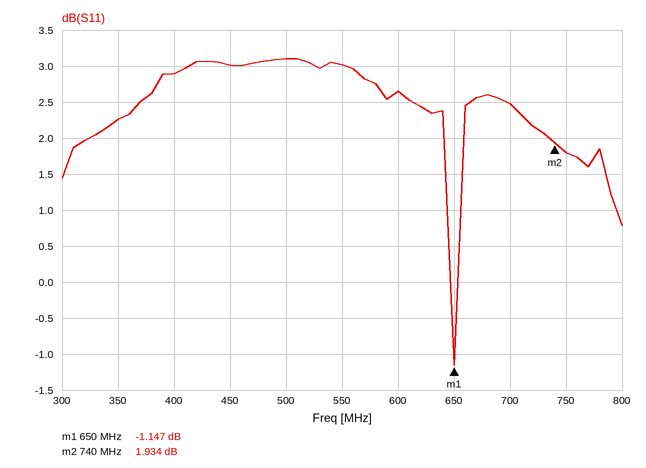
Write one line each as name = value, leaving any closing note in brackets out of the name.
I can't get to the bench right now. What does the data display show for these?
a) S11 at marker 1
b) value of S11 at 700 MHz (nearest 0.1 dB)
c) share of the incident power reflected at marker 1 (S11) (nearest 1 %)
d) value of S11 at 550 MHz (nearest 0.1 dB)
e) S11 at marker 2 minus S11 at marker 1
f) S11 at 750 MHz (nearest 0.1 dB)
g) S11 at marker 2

S11 at marker 1 = -1.147 dB
value of S11 at 700 MHz = 2.5 dB
share of the incident power reflected at marker 1 (S11) = 77 %
value of S11 at 550 MHz = 3.0 dB
S11 at marker 2 minus S11 at marker 1 = 3.081 dB
S11 at 750 MHz = 1.8 dB
S11 at marker 2 = 1.934 dB
